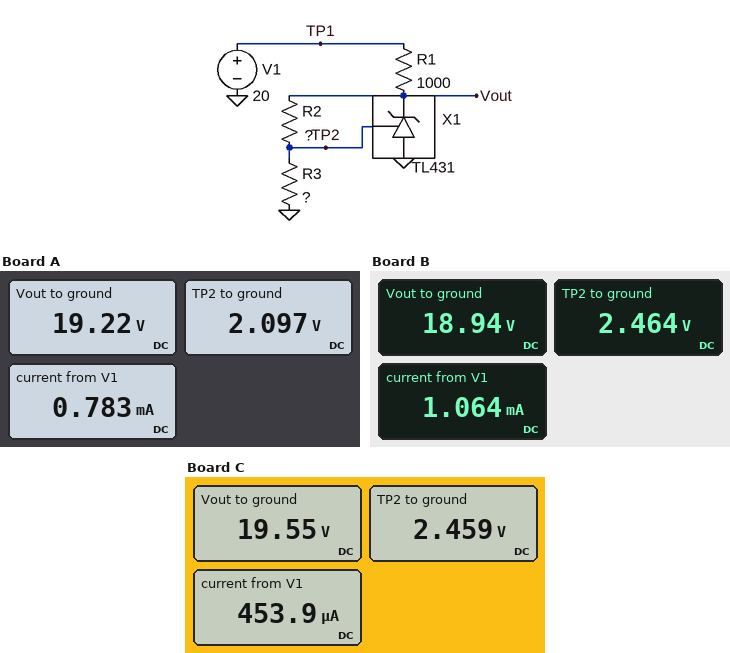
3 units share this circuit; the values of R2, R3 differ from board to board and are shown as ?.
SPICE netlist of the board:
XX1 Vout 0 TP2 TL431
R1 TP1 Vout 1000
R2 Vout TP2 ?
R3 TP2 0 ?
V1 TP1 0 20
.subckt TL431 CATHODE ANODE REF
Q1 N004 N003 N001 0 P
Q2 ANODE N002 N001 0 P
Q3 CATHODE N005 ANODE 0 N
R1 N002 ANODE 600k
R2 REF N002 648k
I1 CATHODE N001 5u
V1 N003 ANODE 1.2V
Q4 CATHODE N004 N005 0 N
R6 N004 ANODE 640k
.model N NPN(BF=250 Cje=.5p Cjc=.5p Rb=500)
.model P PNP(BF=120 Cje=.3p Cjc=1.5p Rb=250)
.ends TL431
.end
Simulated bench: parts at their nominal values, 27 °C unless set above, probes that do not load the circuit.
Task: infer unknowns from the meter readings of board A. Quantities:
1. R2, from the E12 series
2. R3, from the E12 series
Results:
22 kΩ
2.7 kΩ
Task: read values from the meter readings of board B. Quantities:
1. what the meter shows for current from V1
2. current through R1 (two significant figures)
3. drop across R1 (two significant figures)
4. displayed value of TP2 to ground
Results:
1.064 mA
1.1 mA
1.1 V
2.464 V
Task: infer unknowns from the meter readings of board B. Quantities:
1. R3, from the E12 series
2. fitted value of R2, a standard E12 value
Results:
3.3 kΩ
22 kΩ
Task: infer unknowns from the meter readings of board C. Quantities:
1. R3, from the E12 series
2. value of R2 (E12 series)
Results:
6.8 kΩ
47 kΩ
